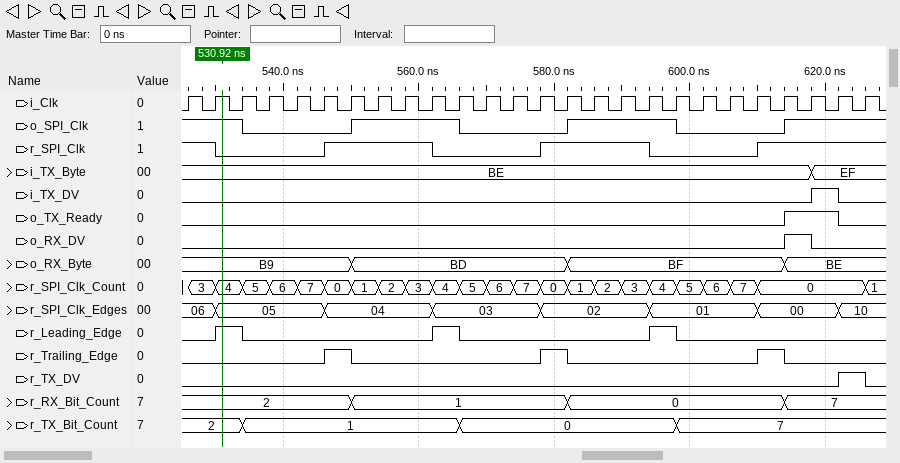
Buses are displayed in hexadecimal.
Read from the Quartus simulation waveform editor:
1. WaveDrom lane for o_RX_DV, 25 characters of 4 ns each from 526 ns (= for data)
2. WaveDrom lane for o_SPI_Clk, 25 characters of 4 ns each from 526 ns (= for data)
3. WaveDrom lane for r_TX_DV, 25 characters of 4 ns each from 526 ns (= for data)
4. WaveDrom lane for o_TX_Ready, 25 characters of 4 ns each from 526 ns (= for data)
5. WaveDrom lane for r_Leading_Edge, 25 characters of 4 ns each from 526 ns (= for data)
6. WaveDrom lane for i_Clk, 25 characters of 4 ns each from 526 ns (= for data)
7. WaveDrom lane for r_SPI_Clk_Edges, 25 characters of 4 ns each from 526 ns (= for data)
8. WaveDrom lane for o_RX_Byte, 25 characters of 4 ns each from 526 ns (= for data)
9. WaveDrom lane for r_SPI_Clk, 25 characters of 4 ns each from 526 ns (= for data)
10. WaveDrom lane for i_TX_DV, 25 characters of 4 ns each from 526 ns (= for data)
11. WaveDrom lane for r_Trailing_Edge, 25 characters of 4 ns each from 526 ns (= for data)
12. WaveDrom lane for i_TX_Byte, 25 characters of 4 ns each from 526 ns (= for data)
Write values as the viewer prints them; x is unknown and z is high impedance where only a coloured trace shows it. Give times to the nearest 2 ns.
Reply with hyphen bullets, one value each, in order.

- {name: 'o_RX_DV', wave: '0.....................10.'}
- {name: 'o_SPI_Clk', wave: '1.0...1...0...1...0...1..'}
- {name: 'r_TX_DV', wave: '0.......................1'}
- {name: 'o_TX_Ready', wave: '0.....................1.0'}
- {name: 'r_Leading_Edge', wave: '010......10......10......'}
- {name: 'i_Clk', wave: 'p........................'}
- {name: 'r_SPI_Clk_Edges', wave: '==...=...=...=...=...=..=', data: '06 05 04 03 02 01 00 10'}
- {name: 'o_RX_Byte', wave: '=.....=.......=.......=..', data: 'B9 BD BF BE'}
- {name: 'r_SPI_Clk', wave: '10...1...0...1...0...1...'}
- {name: 'i_TX_DV', wave: '0......................10'}
- {name: 'r_Trailing_Edge', wave: '0....10......10......10..'}
- {name: 'i_TX_Byte', wave: '=......................=.', data: 'BE EF'}
